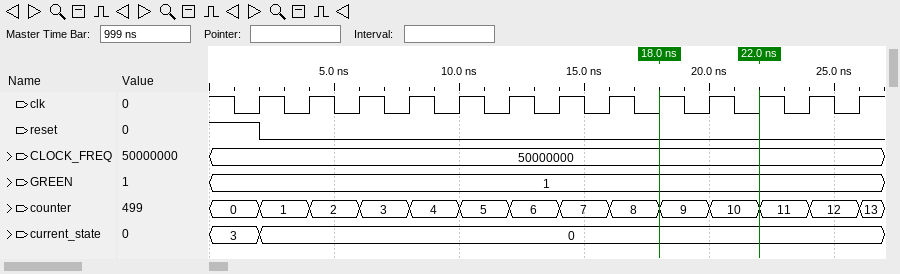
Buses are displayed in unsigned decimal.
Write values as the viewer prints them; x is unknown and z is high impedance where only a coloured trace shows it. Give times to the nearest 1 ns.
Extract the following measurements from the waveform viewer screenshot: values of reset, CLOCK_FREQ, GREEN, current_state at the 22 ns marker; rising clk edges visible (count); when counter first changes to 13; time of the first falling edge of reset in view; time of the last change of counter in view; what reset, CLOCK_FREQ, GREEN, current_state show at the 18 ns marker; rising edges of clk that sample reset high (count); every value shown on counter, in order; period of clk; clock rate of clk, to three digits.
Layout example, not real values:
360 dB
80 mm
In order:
reset=0, CLOCK_FREQ=50000000, GREEN=1, current_state=0
13
26 ns
2 ns
26 ns
reset=0, CLOCK_FREQ=50000000, GREEN=1, current_state=0
1
0, 1, 2, 3, 4, 5, 6, 7, 8, 9, 10, 11, 12, 13
2 ns
500 MHz
